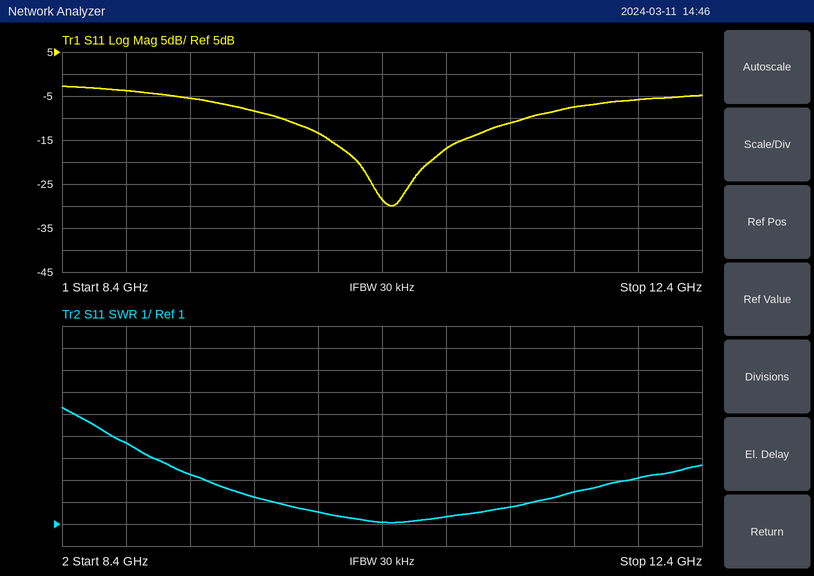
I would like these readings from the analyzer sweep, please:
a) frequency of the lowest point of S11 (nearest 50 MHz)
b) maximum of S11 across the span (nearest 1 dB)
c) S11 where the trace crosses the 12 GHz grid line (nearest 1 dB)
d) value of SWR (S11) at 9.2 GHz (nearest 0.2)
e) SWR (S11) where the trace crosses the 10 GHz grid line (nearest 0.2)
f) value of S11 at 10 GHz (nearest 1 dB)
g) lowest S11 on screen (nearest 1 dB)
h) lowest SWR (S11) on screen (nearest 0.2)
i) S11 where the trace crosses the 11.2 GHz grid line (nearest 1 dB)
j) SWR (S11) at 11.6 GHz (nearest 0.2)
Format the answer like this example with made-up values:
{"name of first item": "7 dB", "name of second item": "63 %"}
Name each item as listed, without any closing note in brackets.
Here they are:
{"frequency of the lowest point of S11": "10.45 GHz", "maximum of S11 across the span": "-3 dB", "S11 where the trace crosses the 12 GHz grid line": "-6 dB", "value of SWR (S11) at 9.2 GHz": "3.2", "SWR (S11) where the trace crosses the 10 GHz grid line": "1.6", "value of S11 at 10 GHz": "-13 dB", "lowest S11 on screen": "-30 dB", "lowest SWR (S11) on screen": "1.0", "S11 where the trace crosses the 11.2 GHz grid line": "-11 dB", "SWR (S11) at 11.6 GHz": "2.4"}
